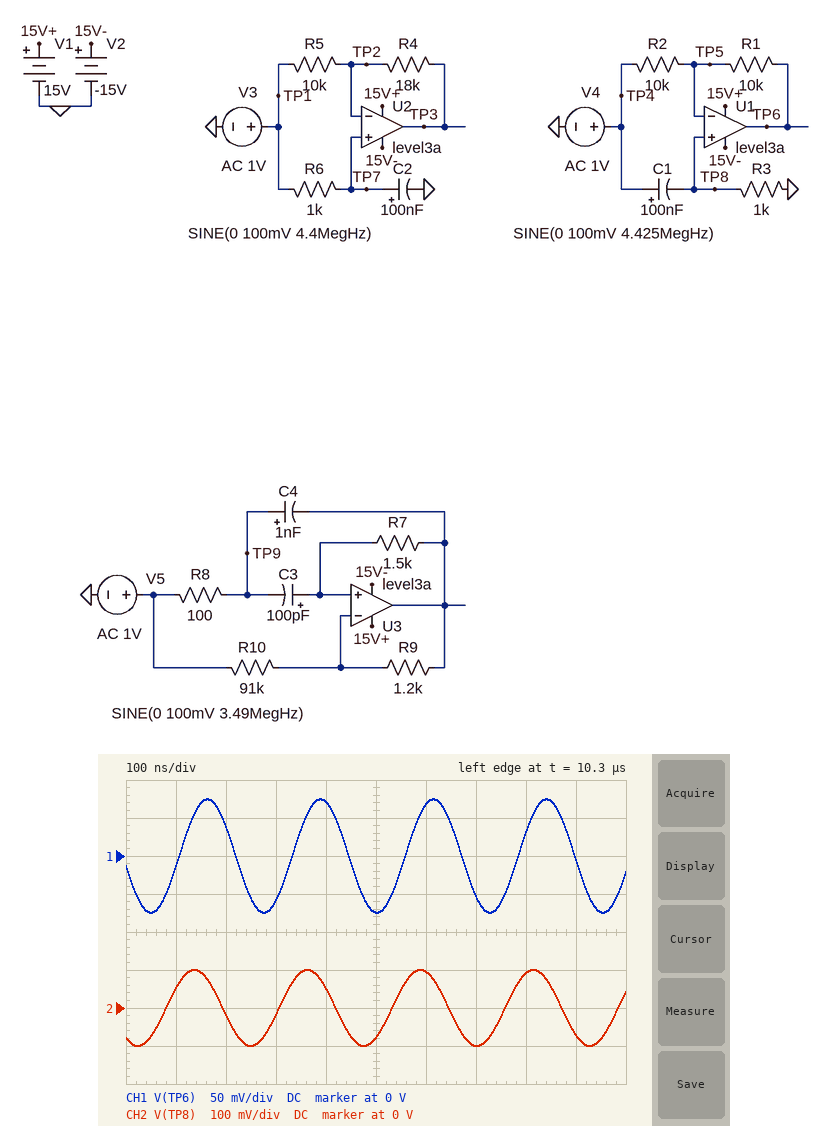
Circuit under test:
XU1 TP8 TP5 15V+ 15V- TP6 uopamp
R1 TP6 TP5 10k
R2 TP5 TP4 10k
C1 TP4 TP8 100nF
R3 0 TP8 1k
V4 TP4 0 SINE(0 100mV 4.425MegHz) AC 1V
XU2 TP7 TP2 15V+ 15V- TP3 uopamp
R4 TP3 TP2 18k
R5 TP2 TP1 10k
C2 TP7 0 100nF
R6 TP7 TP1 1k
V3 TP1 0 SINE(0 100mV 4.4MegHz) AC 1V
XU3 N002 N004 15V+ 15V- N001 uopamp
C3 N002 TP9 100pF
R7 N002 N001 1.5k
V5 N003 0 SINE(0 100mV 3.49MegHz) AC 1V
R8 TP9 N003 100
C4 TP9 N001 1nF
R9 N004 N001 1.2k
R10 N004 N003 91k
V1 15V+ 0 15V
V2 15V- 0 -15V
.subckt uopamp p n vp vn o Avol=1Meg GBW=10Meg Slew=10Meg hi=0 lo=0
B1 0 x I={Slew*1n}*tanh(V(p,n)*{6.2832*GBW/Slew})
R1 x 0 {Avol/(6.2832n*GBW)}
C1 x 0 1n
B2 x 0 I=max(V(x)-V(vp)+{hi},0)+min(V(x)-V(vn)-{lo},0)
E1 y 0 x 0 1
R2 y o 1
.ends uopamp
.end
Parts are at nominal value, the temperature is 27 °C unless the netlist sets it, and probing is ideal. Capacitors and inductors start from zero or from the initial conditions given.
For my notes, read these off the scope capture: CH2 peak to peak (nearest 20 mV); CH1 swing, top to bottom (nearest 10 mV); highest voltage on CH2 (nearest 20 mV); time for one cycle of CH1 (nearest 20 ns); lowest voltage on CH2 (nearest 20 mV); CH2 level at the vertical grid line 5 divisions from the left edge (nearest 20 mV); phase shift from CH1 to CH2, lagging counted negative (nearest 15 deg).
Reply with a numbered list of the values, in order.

1. 200 mV
2. 150 mV
3. 100 mV
4. 220 ns
5. -100 mV
6. -80 mV
7. 45 deg
